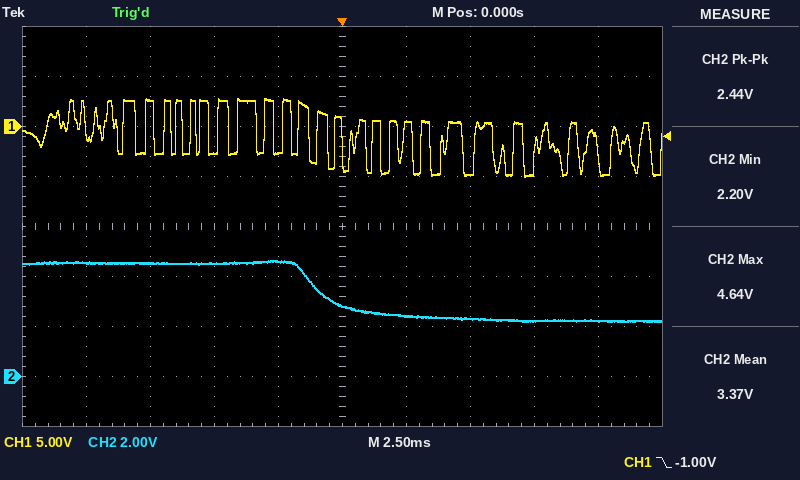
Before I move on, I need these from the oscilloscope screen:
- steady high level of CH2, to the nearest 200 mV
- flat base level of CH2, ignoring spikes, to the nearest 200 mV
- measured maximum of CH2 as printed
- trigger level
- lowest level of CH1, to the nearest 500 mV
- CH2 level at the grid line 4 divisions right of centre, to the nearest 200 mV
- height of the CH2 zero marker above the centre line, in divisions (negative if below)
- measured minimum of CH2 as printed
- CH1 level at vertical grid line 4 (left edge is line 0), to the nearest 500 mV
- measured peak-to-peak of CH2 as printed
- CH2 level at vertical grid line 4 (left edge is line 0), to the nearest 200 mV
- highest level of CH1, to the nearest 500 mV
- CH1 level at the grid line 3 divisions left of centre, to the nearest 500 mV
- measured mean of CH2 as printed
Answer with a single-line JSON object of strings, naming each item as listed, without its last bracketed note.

{"steady high level of CH2, to the nearest 200 mV": "4.6 V", "flat base level of CH2, ignoring spikes, to the nearest 200 mV": "2.2 V", "measured maximum of CH2 as printed": "4.64 V", "trigger level": "-1.00 V", "lowest level of CH1, to the nearest 500 mV": "-5.0 V", "CH2 level at the grid line 4 divisions right of centre, to the nearest 200 mV": "2.2 V", "height of the CH2 zero marker above the centre line, in divisions": "-3.0 div", "measured minimum of CH2 as printed": "2.20 V", "CH1 level at vertical grid line 4 (left edge is line 0), to the nearest 500 mV": "-2.5 V", "measured peak-to-peak of CH2 as printed": "2.44 V", "CH2 level at vertical grid line 4 (left edge is line 0), to the nearest 200 mV": "4.6 V", "highest level of CH1, to the nearest 500 mV": "3.0 V", "CH1 level at the grid line 3 divisions left of centre, to the nearest 500 mV": "2.5 V", "measured mean of CH2 as printed": "3.37 V"}
